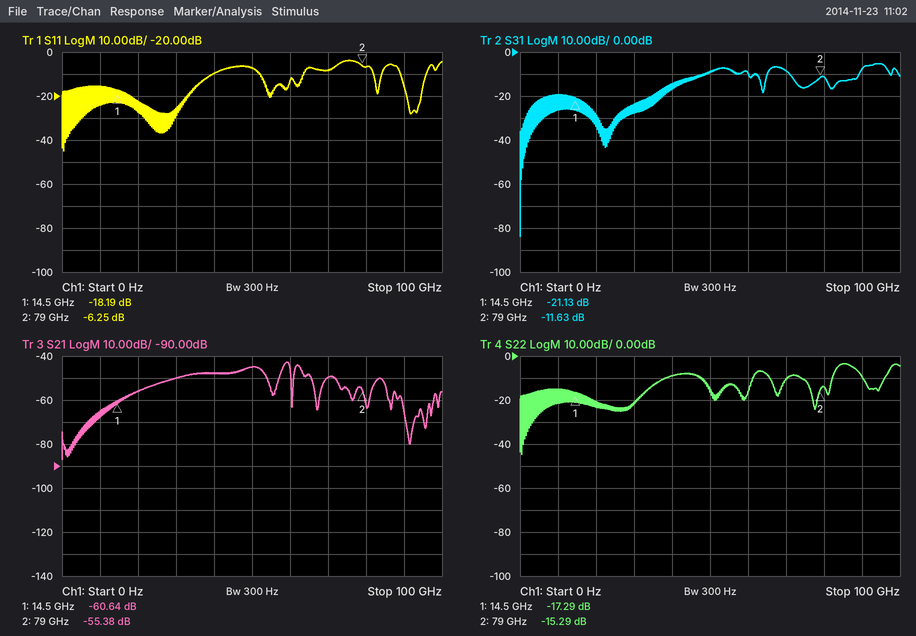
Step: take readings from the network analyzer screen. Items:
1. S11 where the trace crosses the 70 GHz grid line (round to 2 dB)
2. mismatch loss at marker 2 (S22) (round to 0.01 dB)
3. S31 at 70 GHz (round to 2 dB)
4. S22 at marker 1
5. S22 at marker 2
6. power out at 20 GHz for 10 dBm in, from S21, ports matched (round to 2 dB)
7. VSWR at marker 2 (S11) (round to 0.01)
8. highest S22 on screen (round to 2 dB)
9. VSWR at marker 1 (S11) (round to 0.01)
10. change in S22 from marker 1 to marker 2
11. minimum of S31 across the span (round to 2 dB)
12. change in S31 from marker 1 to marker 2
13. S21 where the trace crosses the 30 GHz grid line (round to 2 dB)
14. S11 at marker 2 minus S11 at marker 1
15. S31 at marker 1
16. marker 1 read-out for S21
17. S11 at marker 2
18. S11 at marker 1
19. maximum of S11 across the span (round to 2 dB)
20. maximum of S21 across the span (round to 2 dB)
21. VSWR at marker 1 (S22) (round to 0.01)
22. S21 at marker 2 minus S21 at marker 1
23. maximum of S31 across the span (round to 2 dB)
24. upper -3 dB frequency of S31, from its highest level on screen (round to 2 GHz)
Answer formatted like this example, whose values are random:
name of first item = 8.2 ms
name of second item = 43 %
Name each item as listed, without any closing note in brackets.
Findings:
S11 where the trace crosses the 70 GHz grid line = -8 dB
mismatch loss at marker 2 (S22) = 0.13 dB
S31 at 70 GHz = -8 dB
S22 at marker 1 = -17.29 dB
S22 at marker 2 = -15.29 dB
power out at 20 GHz for 10 dBm in, from S21, ports matched = -46 dBm
VSWR at marker 2 (S11) = 2.90
highest S22 on screen = -4 dB
VSWR at marker 1 (S11) = 1.28
change in S22 from marker 1 to marker 2 = 2.00 dB
minimum of S31 across the span = -84 dB
change in S31 from marker 1 to marker 2 = 9.50 dB
S21 where the trace crosses the 30 GHz grid line = -50 dB
S11 at marker 2 minus S11 at marker 1 = 11.94 dB
S31 at marker 1 = -21.13 dB
marker 1 read-out for S21 = -60.64 dB
S11 at marker 2 = -6.25 dB
S11 at marker 1 = -18.19 dB
maximum of S11 across the span = -4 dB
maximum of S21 across the span = -42 dB
VSWR at marker 1 (S22) = 1.32
S21 at marker 2 minus S21 at marker 1 = 5.26 dB
maximum of S31 across the span = -6 dB
upper -3 dB frequency of S31, from its highest level on screen = 96 GHz
